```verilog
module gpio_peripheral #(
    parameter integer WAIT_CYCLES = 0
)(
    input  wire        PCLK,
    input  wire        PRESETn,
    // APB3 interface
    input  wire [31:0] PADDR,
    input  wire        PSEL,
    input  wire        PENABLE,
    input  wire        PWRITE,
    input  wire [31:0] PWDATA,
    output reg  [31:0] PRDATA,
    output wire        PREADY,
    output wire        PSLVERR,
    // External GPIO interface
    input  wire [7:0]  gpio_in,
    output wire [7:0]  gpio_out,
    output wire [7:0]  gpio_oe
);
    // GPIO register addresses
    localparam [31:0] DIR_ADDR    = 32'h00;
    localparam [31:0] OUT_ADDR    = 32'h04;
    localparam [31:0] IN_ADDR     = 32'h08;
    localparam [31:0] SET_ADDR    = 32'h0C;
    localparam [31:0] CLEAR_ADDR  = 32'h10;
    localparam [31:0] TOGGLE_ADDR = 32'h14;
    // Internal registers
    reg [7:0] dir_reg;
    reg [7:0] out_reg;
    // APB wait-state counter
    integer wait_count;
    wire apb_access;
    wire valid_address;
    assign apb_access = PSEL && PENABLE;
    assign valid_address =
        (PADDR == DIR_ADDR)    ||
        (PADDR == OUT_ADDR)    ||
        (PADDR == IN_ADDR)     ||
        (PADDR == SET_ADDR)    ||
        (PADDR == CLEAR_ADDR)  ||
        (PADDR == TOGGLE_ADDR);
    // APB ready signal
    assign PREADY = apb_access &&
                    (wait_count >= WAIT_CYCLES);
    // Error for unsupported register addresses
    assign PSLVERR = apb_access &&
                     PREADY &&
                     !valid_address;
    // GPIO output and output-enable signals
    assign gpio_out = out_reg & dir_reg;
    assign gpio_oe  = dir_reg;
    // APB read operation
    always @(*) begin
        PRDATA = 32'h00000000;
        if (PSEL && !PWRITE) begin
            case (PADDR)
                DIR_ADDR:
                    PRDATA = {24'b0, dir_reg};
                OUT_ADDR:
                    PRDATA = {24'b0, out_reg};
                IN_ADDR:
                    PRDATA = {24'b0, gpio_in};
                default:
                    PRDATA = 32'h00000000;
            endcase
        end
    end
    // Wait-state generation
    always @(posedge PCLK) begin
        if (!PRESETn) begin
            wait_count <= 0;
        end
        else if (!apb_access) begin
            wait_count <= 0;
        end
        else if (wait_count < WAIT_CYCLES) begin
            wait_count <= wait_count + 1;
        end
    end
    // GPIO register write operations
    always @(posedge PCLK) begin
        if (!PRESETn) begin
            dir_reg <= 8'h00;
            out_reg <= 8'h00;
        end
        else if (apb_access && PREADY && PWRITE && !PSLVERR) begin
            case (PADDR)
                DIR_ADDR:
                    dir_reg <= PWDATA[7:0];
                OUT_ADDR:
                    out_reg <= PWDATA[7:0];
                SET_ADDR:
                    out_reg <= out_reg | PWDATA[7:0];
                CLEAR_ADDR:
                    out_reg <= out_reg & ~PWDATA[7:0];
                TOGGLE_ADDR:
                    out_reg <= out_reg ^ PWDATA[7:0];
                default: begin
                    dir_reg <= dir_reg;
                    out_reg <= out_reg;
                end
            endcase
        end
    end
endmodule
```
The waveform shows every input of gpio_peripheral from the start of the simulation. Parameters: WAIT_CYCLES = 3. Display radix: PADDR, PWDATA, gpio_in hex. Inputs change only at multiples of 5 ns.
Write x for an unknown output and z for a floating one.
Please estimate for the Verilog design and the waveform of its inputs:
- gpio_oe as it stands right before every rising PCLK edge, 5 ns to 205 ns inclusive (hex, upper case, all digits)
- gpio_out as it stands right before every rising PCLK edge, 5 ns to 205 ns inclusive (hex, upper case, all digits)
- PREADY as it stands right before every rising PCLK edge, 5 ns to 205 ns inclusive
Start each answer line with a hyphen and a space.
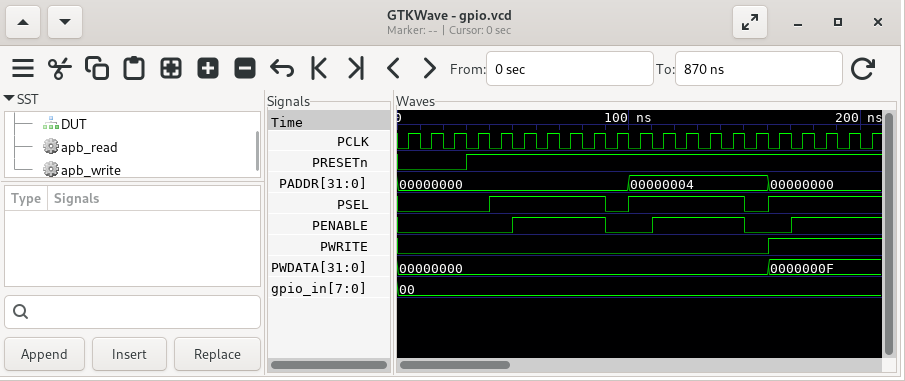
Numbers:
- x, 00, 00, 00, 00, 00, 00, 00, 00, 00, 00, 00, 00, 00, 00, 00, 00, 00, 00, 00, 00
- x, 00, 00, 00, 00, 00, 00, 00, 00, 00, 00, 00, 00, 00, 00, 00, 00, 00, 00, 00, 00
- 0 0 0 0 0 0 0 0 1 0 0 0 0 0 1 0 0 0 0 0 1
